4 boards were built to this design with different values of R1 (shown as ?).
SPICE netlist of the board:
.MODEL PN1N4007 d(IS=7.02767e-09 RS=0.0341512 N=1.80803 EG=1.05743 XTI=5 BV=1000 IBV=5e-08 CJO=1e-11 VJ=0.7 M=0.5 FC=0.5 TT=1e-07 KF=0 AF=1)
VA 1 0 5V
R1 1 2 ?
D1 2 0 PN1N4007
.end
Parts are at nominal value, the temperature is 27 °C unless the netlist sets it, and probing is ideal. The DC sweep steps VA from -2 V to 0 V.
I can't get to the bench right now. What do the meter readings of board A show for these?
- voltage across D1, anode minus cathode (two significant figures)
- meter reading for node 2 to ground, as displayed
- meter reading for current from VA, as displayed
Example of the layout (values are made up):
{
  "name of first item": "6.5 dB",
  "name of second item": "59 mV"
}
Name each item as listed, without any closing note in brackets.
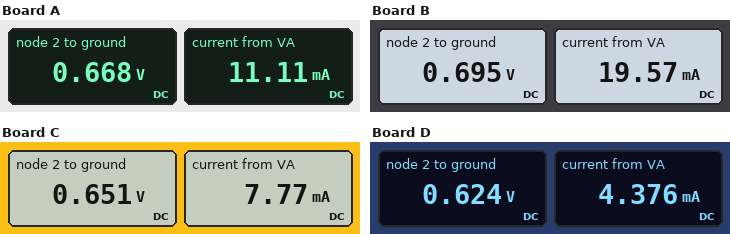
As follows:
{
  "voltage across D1, anode minus cathode": "670 mV",
  "meter reading for node 2 to ground, as displayed": "0.668 V",
  "meter reading for current from VA, as displayed": "11.11 mA"
}
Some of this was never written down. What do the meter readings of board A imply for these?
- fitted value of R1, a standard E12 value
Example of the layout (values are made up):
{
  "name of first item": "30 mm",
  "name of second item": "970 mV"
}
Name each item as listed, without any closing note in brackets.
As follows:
{
  "fitted value of R1, a standard E12 value": "390 Ω"
}
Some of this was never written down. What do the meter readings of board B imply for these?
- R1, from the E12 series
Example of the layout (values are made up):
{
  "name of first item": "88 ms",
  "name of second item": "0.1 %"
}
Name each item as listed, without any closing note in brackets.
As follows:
{
  "R1, from the E12 series": "220 Ω"
}
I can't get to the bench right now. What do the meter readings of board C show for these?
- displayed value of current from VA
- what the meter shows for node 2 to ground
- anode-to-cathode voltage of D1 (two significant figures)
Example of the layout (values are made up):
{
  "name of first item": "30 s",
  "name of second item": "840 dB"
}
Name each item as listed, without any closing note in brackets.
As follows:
{
  "displayed value of current from VA": "7.77 mA",
  "what the meter shows for node 2 to ground": "0.651 V",
  "anode-to-cathode voltage of D1": "650 mV"
}
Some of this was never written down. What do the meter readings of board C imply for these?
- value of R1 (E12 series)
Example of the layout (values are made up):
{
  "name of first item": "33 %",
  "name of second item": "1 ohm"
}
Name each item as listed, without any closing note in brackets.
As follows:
{
  "value of R1": "560 Ω"
}
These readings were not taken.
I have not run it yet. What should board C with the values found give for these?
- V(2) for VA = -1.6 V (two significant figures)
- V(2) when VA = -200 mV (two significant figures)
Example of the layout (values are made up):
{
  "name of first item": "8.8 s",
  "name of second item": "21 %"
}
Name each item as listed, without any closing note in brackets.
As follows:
{
  "V(2) for VA = -1.6 V": "-1.6 V",
  "V(2) when VA = -200 mV": "-200 mV"
}
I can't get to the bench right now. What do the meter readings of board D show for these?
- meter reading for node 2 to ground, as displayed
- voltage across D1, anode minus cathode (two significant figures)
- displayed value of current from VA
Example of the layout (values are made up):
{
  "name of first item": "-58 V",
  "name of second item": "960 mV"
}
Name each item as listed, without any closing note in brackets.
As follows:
{
  "meter reading for node 2 to ground, as displayed": "0.624 V",
  "voltage across D1, anode minus cathode": "620 mV",
  "displayed value of current from VA": "4.376 mA"
}
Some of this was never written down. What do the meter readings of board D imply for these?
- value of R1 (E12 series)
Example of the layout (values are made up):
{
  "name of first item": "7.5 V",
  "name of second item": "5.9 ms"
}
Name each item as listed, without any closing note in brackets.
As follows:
{
  "value of R1": "1 kΩ"
}
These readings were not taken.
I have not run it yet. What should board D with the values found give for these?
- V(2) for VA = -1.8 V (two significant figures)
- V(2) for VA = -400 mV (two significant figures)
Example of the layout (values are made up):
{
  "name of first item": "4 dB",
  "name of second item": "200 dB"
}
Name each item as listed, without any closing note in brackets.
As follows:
{
  "V(2) for VA = -1.8 V": "-1.8 V",
  "V(2) for VA = -400 mV": "-400 mV"
}
